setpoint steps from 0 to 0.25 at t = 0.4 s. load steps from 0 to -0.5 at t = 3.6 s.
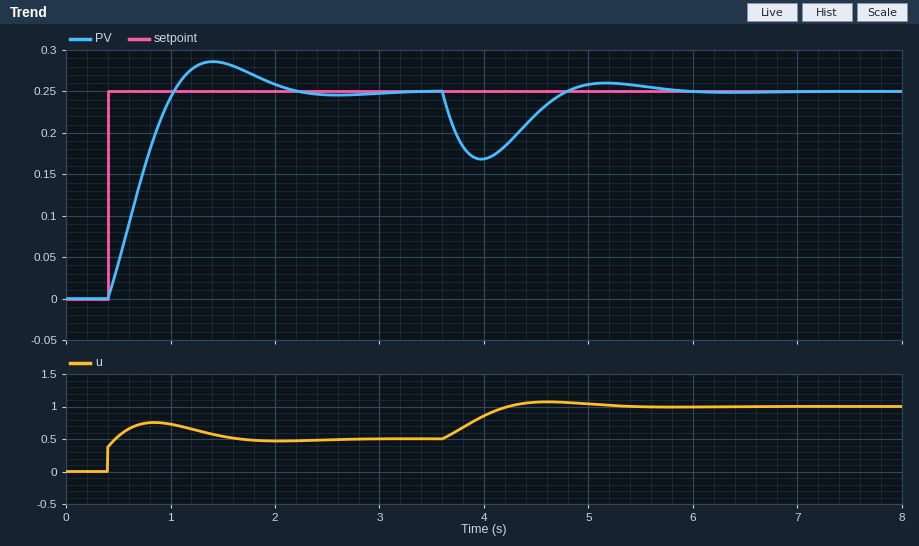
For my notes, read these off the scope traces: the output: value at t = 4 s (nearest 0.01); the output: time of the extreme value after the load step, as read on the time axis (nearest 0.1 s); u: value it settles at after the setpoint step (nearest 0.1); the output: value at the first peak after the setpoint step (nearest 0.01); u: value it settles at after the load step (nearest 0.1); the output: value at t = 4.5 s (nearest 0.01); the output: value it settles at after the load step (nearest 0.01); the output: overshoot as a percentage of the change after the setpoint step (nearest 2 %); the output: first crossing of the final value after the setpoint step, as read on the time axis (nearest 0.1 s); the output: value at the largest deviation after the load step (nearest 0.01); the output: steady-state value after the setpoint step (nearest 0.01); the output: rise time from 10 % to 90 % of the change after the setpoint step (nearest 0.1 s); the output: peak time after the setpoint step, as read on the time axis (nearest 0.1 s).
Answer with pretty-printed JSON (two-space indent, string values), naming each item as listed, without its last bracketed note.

{
  "the output: value at t = 4 s": "0.17",
  "the output: time of the extreme value after the load step, as read on the time axis": "4.0 s",
  "u: value it settles at after the setpoint step": "0.5",
  "the output: value at the first peak after the setpoint step": "0.29",
  "u: value it settles at after the load step": "1.0",
  "the output: value at t = 4.5 s": "0.22",
  "the output: value it settles at after the load step": "0.25",
  "the output: overshoot as a percentage of the change after the setpoint step": "14 %",
  "the output: first crossing of the final value after the setpoint step, as read on the time axis": "1.0 s",
  "the output: value at the largest deviation after the load step": "0.17",
  "the output: steady-state value after the setpoint step": "0.25",
  "the output: rise time from 10 % to 90 % of the change after the setpoint step": "0.5 s",
  "the output: peak time after the setpoint step, as read on the time axis": "1.4 s"
}
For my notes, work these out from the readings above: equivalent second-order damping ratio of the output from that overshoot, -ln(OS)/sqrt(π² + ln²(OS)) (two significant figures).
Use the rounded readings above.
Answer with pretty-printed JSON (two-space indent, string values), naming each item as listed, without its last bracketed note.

{
  "equivalent second-order damping ratio of the output from that overshoot, -ln(OS)/sqrt(π² + ln²(OS))": "0.53"
}
